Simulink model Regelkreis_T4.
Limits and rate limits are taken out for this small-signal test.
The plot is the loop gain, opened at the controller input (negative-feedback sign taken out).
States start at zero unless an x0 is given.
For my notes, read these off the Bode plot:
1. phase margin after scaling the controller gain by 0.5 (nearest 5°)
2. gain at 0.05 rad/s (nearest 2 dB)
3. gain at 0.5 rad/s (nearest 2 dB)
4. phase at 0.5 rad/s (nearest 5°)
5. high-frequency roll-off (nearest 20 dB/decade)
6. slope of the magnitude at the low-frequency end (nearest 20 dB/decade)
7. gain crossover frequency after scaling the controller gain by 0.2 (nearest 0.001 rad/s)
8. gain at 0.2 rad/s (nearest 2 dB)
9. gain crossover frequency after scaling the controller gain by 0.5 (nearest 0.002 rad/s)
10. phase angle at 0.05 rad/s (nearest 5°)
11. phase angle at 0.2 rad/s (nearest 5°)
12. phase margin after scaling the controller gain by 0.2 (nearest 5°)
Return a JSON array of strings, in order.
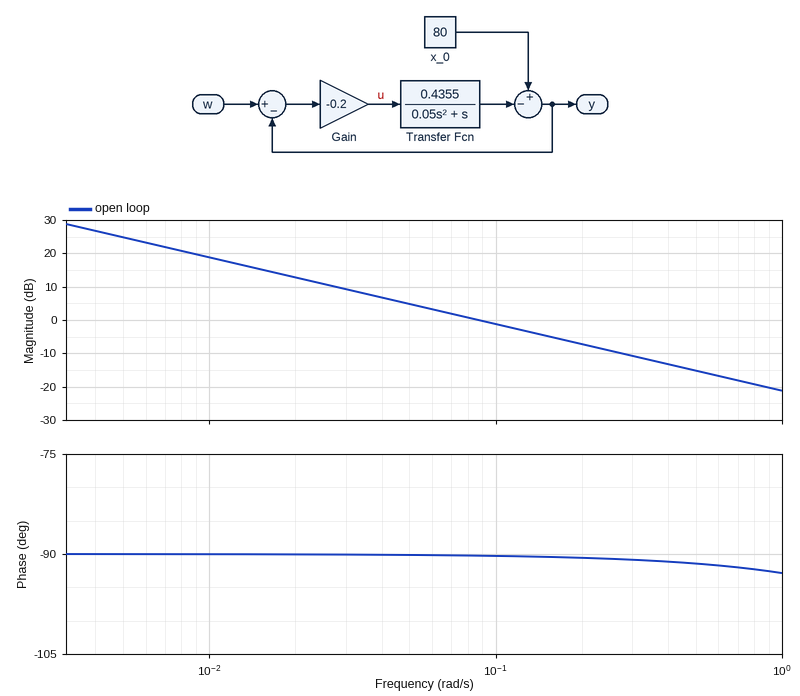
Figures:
["90°", "4 dB", "-16 dB", "-90°", "-20 dB/decade", "-20 dB/decade", "0.017 rad/s", "-8 dB", "0.044 rad/s", "-90°", "-90°", "90°"]
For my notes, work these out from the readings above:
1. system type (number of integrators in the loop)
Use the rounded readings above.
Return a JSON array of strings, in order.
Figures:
["1"]
